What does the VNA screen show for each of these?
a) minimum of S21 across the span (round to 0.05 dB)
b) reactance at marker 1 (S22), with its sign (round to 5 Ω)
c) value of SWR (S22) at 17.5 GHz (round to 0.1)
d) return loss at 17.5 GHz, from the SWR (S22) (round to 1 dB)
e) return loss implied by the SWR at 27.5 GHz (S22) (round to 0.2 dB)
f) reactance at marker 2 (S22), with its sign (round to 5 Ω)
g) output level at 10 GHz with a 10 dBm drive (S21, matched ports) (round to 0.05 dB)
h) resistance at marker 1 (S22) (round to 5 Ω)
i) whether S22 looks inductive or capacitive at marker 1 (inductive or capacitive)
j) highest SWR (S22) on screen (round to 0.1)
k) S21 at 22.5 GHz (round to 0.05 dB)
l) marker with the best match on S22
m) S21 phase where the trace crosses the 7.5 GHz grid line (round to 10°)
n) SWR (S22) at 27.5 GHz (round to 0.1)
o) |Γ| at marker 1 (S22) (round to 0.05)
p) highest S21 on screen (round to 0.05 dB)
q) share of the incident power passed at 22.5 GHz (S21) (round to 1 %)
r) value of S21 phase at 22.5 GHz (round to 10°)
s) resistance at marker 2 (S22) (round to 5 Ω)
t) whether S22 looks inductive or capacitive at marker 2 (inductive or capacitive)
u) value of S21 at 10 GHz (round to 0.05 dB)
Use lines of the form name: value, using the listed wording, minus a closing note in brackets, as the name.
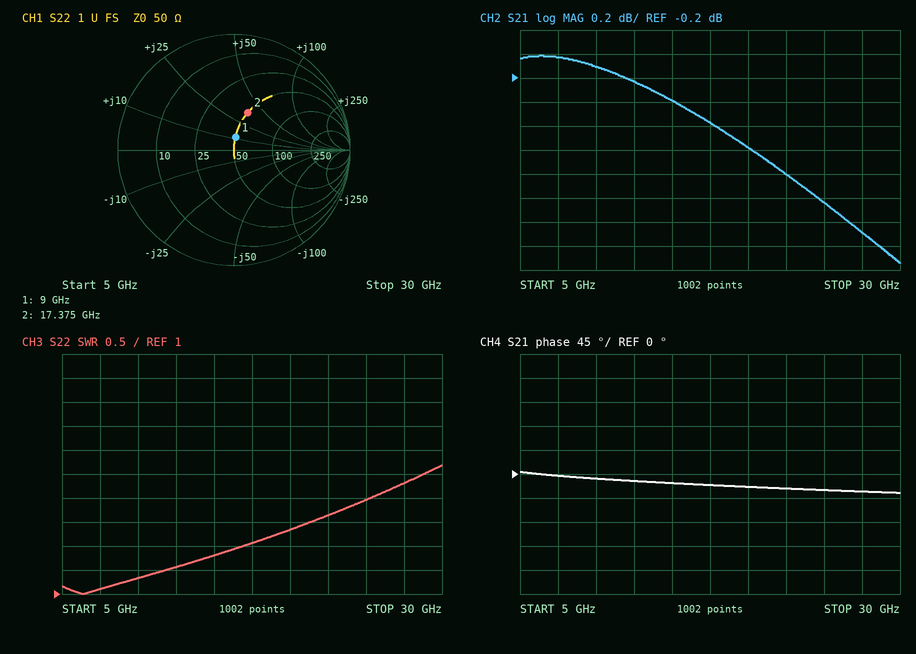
minimum of S21 across the span: -1.75 dB
reactance at marker 1 (S22), with its sign: +10 Ω
value of SWR (S22) at 17.5 GHz: 2.1
return loss at 17.5 GHz, from the SWR (S22): 9 dB
return loss implied by the SWR at 27.5 GHz (S22): 5.4 dB
reactance at marker 2 (S22), with its sign: +35 Ω
output level at 10 GHz with a 10 dBm drive (S21, matched ports): 9.90 dBm
resistance at marker 1 (S22): 50 Ω
whether S22 looks inductive or capacitive at marker 1: inductive
highest SWR (S22) on screen: 3.7
S21 at 22.5 GHz: -1.00 dB
marker with the best match on S22: marker 1
S21 phase where the trace crosses the 7.5 GHz grid line: 0°
SWR (S22) at 27.5 GHz: 3.3
|Γ| at marker 1 (S22): 0.10
highest S21 on screen: 0.00 dB
share of the incident power passed at 22.5 GHz (S21): 79 %
value of S21 phase at 22.5 GHz: -30°
resistance at marker 2 (S22): 50 Ω
whether S22 looks inductive or capacitive at marker 2: inductive
value of S21 at 10 GHz: -0.10 dB
